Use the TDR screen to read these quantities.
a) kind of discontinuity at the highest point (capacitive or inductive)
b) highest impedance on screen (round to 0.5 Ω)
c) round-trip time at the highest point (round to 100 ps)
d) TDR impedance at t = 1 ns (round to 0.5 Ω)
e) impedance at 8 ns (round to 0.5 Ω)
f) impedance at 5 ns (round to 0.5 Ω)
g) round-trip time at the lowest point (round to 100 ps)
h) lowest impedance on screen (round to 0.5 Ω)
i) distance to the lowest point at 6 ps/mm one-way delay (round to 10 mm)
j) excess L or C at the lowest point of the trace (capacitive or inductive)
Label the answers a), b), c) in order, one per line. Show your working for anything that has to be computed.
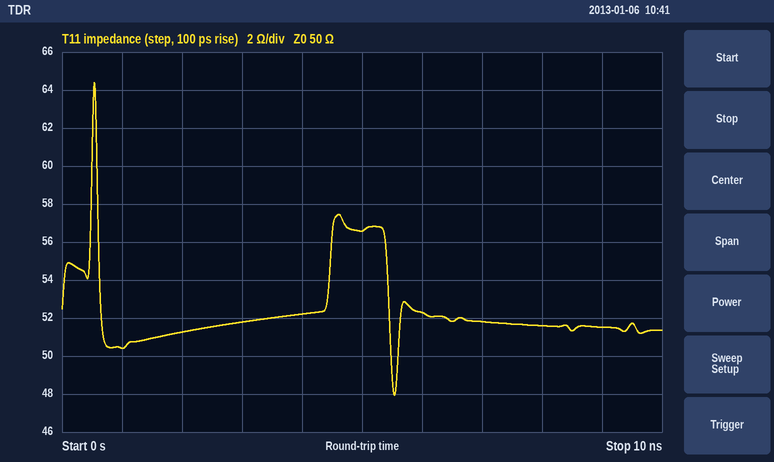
a) inductive
b) 64.5 Ω
c) 500 ps
d) 50.5 Ω
e) 51.5 Ω
f) 56.5 Ω
g) 5.5 ns
h) 48.0 Ω
i) 5.5 ns / 2 / 6 ps/mm ≈ 458 mm, so 460 mm to the nearest 10 mm
j) capacitive
